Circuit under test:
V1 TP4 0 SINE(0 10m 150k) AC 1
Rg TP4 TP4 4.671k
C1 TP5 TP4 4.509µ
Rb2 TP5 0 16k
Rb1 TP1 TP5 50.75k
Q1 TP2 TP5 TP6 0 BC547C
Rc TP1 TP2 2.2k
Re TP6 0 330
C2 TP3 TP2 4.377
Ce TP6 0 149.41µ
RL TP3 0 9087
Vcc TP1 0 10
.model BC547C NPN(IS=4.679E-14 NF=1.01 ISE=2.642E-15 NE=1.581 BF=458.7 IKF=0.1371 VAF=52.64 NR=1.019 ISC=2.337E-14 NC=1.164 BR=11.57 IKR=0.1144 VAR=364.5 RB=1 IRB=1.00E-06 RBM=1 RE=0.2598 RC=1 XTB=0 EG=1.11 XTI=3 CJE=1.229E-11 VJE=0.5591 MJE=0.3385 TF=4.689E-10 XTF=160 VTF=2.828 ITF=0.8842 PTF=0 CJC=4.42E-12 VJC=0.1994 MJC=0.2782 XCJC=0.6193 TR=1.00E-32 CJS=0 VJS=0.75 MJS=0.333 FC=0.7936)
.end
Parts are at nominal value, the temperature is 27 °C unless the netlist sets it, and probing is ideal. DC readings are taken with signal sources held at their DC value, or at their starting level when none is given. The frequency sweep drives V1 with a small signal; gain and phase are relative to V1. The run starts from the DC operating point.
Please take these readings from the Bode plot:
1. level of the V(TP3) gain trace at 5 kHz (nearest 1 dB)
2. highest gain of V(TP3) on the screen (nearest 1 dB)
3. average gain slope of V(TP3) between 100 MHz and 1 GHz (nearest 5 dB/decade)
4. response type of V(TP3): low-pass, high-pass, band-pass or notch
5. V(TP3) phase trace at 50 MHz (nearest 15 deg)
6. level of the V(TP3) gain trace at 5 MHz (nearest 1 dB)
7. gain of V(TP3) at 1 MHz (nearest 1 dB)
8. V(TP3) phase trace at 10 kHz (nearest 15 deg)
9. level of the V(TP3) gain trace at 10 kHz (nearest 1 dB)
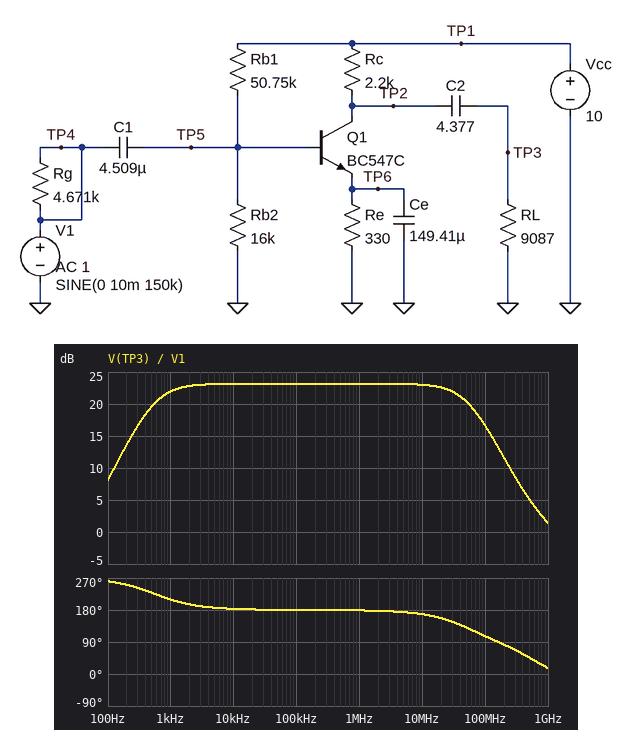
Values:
23 dB
23 dB
-15 dB/decade
band-pass
135 deg
23 dB
23 dB
180 deg
23 dB
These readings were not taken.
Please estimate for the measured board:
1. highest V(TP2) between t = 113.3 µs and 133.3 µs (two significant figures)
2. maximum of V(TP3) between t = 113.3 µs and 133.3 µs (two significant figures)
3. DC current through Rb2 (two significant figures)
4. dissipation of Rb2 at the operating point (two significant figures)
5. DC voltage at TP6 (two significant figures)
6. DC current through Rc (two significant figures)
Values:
3.2 V
1.8 V
120 µA
240 µW
1.3 V
3.9 mA
